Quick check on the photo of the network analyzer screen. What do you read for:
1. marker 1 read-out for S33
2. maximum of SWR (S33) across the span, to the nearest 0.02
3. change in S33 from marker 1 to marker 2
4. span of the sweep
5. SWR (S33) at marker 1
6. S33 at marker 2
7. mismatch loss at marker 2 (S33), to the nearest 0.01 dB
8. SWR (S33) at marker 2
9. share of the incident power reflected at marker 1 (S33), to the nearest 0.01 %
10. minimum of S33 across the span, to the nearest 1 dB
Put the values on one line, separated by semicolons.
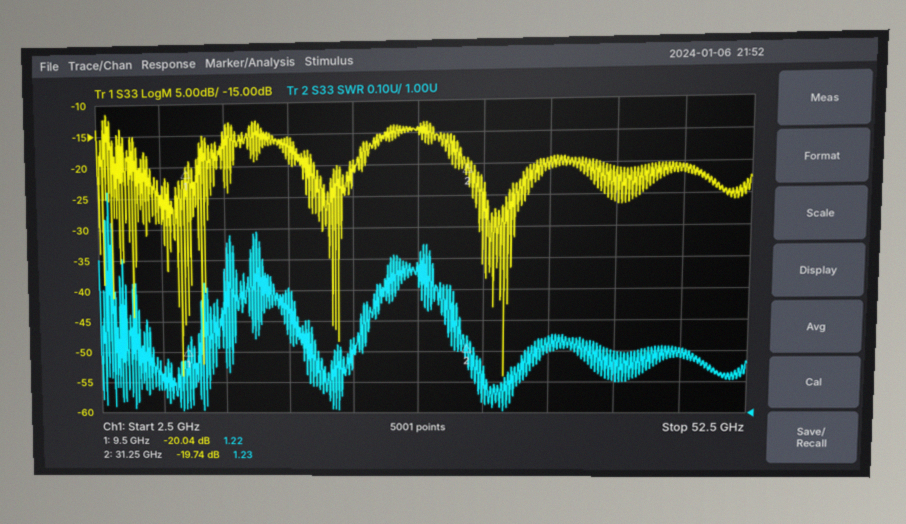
-20.04 dB; 1.72; 0.30 dB; 50 GHz; 1.22; -19.74 dB; 0.05 dB; 1.23; 0.99 %; -54 dB
